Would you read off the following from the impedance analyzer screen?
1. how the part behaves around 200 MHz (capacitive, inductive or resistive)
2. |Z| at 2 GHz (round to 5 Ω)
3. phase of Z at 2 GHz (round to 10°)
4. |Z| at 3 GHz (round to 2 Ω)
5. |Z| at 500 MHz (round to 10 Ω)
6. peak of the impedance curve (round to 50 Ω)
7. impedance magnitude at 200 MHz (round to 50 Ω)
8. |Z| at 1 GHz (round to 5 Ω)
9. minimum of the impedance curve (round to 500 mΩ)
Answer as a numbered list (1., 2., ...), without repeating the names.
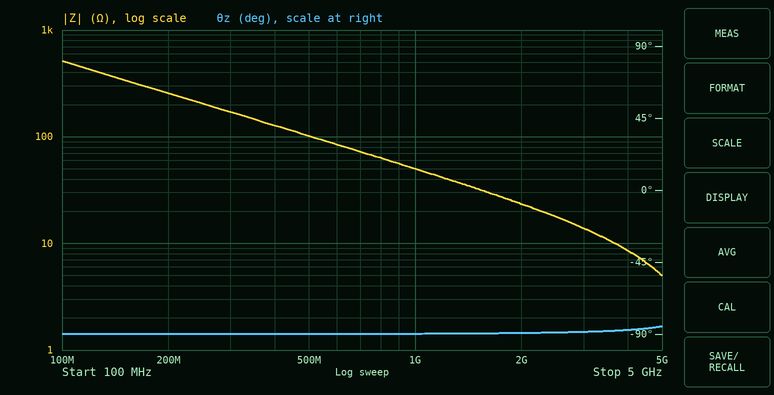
1. capacitive
2. 25 Ω
3. -90°
4. 14 Ω
5. 100 Ω
6. 500 Ω
7. 250 Ω
8. 50 Ω
9. 5.0 Ω
